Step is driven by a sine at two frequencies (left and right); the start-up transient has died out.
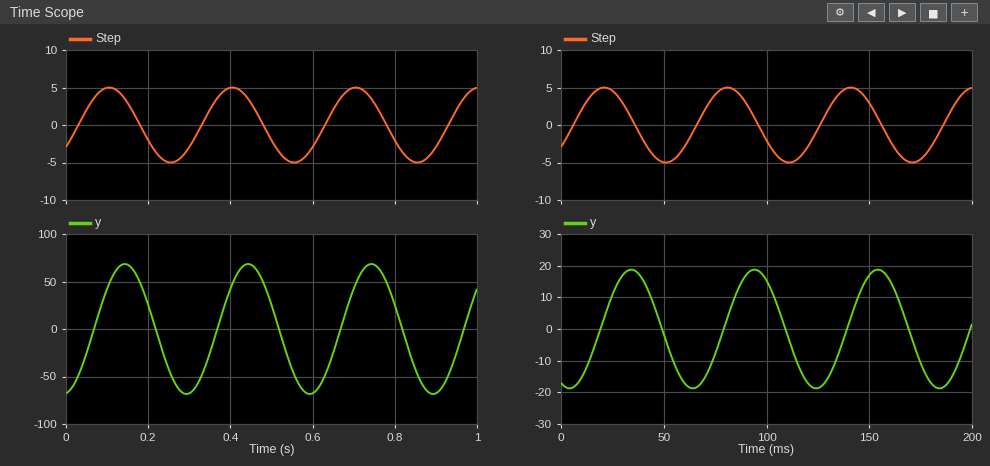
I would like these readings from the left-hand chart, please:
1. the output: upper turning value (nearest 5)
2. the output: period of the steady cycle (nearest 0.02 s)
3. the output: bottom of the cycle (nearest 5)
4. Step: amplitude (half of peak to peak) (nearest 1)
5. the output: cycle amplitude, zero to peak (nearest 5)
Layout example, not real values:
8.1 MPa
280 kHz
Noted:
70
0.30 s
-70
5
70
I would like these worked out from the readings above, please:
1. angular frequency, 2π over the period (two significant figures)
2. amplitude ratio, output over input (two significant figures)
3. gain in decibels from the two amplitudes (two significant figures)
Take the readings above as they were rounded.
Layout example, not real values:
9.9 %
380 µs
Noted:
21 rad/s
14
23 dB
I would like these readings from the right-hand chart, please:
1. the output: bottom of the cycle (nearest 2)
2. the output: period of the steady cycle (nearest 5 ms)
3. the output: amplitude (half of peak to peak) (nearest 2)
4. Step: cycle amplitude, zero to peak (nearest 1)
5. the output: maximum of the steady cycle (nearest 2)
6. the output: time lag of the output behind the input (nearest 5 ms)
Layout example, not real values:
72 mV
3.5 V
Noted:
-18
60 ms
18
5
18
15 ms
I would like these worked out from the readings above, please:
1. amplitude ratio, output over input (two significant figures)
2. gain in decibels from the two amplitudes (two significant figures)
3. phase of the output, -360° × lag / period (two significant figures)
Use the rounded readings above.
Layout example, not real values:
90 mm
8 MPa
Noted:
3.6
11 dB
-90°
